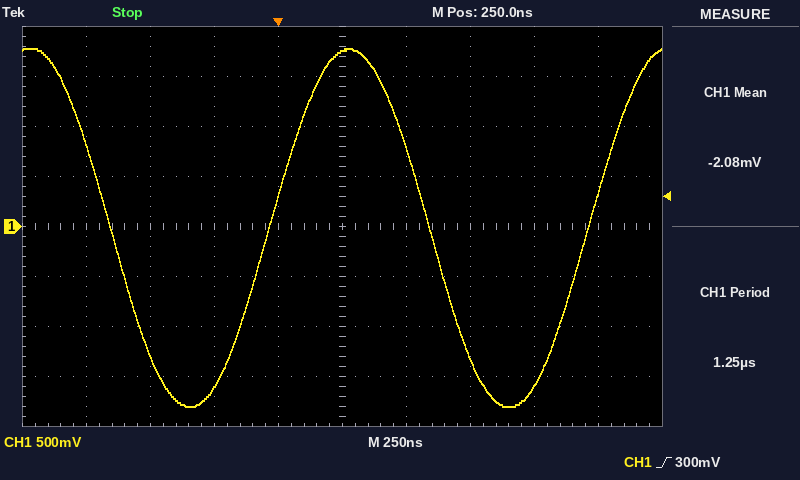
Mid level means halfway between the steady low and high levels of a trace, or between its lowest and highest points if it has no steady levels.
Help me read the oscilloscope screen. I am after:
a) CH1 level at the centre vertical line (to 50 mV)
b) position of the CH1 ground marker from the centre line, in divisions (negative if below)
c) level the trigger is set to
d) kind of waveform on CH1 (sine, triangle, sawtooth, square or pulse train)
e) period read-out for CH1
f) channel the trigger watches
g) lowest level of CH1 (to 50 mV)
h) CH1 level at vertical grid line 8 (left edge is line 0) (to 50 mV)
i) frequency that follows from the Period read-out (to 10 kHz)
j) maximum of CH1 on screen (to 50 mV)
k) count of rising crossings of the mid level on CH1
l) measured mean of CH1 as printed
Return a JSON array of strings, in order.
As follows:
["1.75 V", "0.0 div", "300 mV", "sine", "1.25 µs", "CH1", "-1.80 V", "-1.60 V", "800 kHz", "1.80 V", "2", "-2.08 mV"]
